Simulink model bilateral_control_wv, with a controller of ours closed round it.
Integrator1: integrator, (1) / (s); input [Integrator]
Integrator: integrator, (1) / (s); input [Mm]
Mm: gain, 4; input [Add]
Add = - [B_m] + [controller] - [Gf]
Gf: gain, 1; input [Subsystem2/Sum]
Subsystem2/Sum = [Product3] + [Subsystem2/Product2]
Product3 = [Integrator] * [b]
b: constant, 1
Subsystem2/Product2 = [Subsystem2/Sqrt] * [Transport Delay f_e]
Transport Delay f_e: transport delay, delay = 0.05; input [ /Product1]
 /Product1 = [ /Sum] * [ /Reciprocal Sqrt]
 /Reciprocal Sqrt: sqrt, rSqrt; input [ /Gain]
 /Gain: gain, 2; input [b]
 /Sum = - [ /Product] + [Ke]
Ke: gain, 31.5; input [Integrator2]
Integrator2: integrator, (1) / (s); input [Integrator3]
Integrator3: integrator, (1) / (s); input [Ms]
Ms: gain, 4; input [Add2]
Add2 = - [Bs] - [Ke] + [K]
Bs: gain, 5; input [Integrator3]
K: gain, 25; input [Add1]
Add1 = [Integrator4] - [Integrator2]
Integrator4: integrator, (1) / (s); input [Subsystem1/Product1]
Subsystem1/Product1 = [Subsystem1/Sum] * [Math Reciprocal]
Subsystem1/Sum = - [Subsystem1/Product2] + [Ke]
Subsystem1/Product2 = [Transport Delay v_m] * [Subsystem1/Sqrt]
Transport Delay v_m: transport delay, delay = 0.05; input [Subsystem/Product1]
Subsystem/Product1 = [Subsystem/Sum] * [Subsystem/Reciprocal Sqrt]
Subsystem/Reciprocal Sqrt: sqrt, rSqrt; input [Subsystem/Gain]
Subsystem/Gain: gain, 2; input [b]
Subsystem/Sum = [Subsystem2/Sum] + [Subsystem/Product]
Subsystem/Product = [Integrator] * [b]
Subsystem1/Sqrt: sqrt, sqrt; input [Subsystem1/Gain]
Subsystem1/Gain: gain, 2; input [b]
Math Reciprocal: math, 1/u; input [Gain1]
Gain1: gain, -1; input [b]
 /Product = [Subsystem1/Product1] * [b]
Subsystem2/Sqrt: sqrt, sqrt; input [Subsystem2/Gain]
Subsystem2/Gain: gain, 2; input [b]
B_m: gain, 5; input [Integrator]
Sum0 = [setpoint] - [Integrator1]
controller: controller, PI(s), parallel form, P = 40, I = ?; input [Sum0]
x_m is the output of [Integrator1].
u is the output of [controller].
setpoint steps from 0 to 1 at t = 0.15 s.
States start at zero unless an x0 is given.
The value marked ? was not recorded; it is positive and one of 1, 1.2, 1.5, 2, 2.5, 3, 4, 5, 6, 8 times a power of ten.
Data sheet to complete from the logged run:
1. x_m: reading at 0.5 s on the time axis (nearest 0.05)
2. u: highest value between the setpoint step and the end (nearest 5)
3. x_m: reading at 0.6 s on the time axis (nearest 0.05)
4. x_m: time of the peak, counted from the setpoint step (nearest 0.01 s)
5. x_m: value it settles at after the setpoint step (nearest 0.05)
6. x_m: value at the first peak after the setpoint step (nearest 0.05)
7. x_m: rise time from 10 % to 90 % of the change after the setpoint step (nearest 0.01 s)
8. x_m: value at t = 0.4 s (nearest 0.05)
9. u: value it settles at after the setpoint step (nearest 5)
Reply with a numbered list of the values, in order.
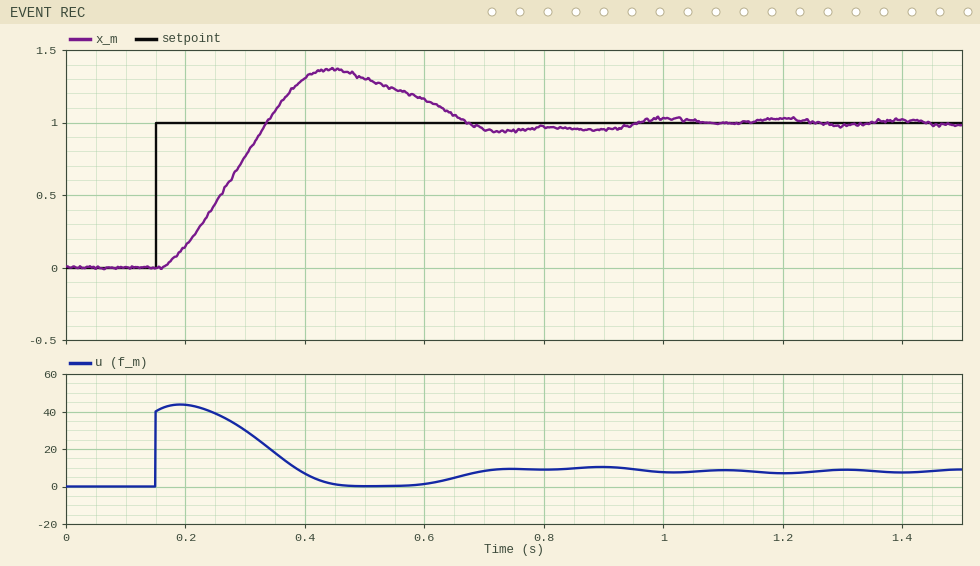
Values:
1. 1.30
2. 45
3. 1.15
4. 0.29 s
5. 1.00
6. 1.35
7. 0.13 s
8. 1.30
9. 10
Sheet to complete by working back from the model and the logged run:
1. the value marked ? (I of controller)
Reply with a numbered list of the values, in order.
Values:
1. 200
